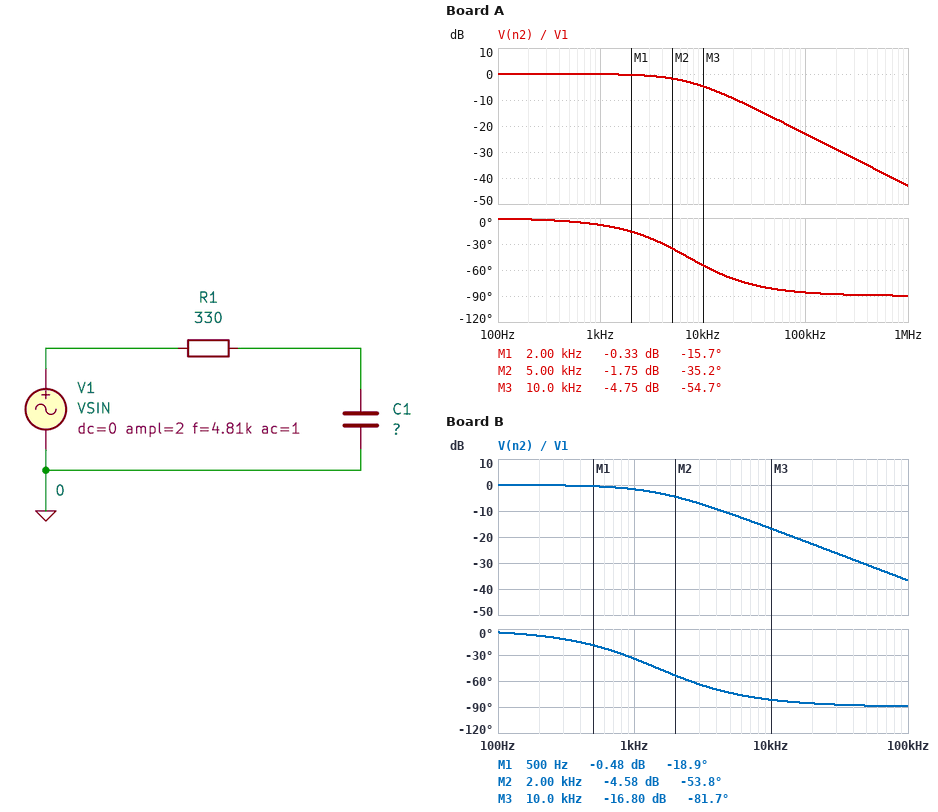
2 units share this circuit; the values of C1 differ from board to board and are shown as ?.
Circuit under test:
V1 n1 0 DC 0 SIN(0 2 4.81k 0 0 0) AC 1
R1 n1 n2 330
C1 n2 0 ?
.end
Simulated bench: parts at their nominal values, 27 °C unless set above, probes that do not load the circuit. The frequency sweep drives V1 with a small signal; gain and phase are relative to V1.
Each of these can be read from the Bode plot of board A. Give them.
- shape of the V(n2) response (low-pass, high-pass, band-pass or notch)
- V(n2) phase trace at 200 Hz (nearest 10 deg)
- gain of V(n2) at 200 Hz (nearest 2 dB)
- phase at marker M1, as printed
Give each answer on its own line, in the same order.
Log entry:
low-pass
0 deg
0 dB
-15.7 deg
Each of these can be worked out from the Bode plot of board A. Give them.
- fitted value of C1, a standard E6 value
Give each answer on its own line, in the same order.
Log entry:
68 nF
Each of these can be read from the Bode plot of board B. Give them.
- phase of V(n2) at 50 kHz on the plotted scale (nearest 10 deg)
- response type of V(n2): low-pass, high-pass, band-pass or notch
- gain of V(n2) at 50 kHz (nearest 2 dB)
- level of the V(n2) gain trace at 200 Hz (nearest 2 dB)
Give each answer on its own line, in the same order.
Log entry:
-90 deg
low-pass
-30 dB
0 dB
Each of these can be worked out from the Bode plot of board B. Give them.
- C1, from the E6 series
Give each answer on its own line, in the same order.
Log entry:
330 nF
